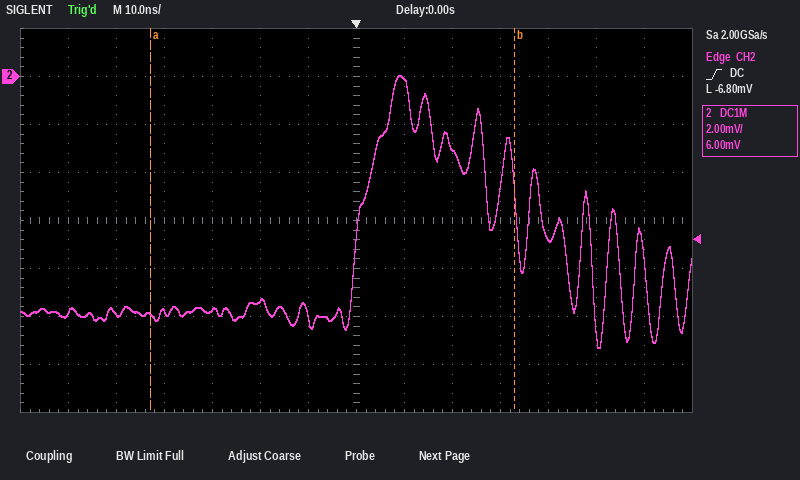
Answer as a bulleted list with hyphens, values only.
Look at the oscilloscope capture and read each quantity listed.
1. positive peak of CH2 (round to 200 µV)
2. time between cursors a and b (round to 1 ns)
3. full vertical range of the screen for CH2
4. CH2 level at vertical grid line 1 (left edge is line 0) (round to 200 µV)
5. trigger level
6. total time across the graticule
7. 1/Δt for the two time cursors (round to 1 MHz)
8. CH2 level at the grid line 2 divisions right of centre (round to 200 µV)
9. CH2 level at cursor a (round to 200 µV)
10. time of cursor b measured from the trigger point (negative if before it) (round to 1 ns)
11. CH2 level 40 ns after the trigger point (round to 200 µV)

- 0.0 mV
- 76 ns
- 16 mV
- -9.8 mV
- -6.80 mV
- 140 ns
- 13 MHz
- -3.0 mV
- -10.0 mV
- +33 ns
- -6.8 mV
